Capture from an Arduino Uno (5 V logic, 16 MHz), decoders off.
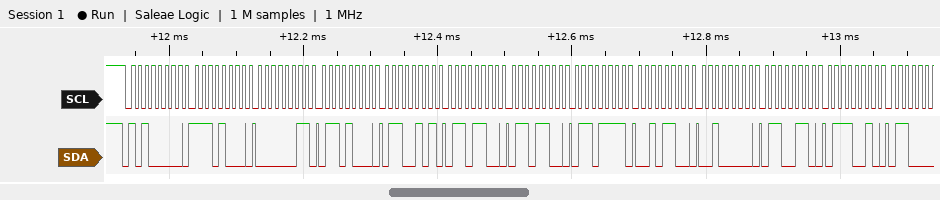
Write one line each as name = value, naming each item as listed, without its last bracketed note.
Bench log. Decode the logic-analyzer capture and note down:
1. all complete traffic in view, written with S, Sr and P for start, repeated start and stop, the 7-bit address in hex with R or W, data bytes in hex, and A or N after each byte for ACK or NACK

all complete traffic in view, written with S, Sr and P for start, repeated start and stop, the 7-bit address in hex with R or W, data bytes in hex, and A or N after each byte for ACK or NACK = S 50W A E8 A 03 A 68 A 65 A 6C A 6C A 6F A 2C A 20 A 66 A 72 A
